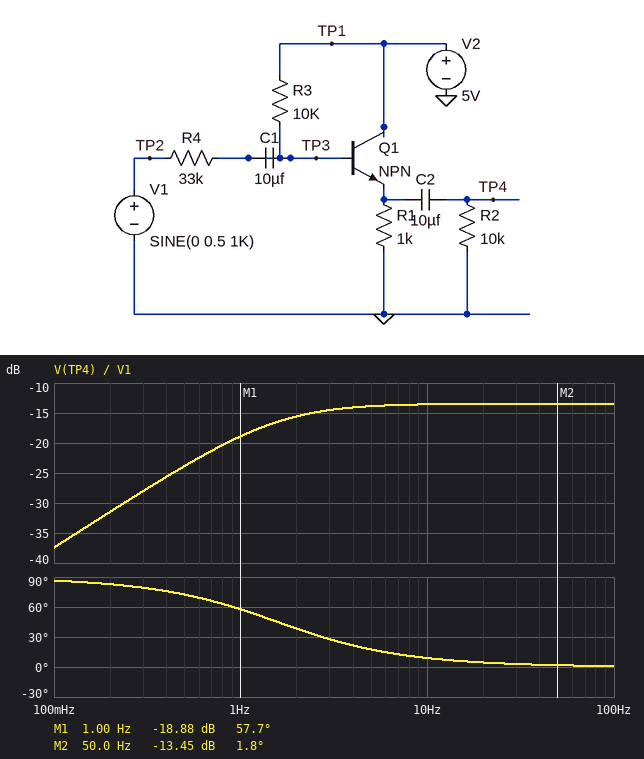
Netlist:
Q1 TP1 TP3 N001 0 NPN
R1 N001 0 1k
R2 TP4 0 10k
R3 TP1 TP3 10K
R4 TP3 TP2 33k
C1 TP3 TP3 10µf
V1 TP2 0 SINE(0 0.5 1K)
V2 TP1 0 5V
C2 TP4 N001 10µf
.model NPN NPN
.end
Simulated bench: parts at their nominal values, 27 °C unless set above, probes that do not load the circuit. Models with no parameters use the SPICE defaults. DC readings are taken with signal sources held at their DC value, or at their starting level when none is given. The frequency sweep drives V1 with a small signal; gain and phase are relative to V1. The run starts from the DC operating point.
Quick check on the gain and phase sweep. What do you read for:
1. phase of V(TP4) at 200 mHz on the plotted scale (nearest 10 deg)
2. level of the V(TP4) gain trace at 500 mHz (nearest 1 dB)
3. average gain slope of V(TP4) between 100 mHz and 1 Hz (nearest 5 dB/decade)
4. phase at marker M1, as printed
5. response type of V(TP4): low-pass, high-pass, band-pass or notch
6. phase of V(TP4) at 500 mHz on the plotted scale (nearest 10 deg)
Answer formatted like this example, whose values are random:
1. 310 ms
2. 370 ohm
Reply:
1. 80 deg
2. -24 dB
3. 20 dB/decade
4. 57.7 deg
5. high-pass
6. 70 deg
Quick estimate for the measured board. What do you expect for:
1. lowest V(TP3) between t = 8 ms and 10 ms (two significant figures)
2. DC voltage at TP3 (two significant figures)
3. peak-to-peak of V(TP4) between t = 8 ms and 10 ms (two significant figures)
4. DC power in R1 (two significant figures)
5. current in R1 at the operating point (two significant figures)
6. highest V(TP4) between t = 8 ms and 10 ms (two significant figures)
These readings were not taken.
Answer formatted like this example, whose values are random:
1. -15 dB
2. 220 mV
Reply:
1. 3.5 V
2. 3.6 V
3. 210 mV
4. 8.0 mW
5. 2.8 mA
6. 110 mV
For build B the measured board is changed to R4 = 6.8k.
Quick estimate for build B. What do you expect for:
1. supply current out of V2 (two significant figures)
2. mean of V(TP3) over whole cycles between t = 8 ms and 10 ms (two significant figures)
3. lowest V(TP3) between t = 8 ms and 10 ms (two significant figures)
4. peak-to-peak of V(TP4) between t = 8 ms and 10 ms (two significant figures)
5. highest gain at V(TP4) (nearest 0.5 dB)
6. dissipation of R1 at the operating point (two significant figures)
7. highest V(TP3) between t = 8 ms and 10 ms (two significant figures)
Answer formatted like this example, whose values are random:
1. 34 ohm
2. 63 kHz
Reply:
1. 1.5 mA
2. 2.0 V
3. 1.7 V
4. 560 mV
5. -5.0 dB
6. 1.4 mW
7. 2.3 V
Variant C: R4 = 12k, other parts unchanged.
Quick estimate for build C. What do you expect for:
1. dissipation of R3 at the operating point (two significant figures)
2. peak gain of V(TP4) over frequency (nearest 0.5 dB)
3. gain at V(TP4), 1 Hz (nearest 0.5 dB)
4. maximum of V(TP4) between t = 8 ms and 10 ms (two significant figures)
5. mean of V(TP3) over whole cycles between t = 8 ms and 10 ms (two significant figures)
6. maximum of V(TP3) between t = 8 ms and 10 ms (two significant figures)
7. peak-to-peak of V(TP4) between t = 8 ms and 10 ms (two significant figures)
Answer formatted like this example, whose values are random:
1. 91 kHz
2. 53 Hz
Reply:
1. 560 µW
2. -7.5 dB
3. -13.0 dB
4. 210 mV
5. 2.6 V
6. 2.8 V
7. 420 mV
